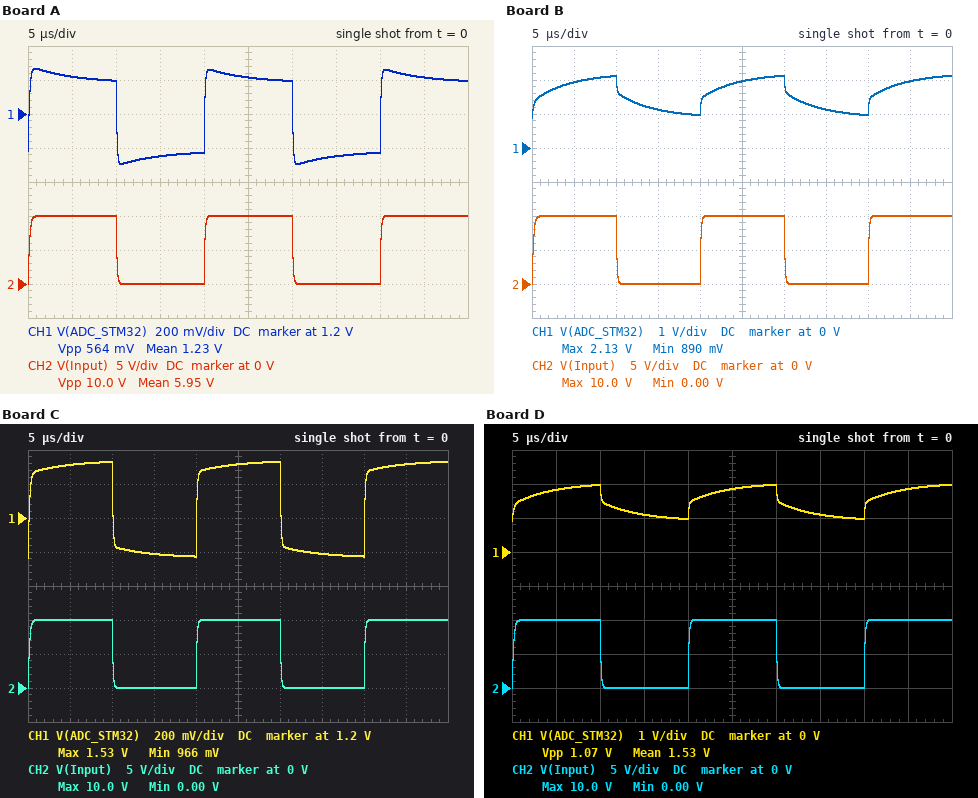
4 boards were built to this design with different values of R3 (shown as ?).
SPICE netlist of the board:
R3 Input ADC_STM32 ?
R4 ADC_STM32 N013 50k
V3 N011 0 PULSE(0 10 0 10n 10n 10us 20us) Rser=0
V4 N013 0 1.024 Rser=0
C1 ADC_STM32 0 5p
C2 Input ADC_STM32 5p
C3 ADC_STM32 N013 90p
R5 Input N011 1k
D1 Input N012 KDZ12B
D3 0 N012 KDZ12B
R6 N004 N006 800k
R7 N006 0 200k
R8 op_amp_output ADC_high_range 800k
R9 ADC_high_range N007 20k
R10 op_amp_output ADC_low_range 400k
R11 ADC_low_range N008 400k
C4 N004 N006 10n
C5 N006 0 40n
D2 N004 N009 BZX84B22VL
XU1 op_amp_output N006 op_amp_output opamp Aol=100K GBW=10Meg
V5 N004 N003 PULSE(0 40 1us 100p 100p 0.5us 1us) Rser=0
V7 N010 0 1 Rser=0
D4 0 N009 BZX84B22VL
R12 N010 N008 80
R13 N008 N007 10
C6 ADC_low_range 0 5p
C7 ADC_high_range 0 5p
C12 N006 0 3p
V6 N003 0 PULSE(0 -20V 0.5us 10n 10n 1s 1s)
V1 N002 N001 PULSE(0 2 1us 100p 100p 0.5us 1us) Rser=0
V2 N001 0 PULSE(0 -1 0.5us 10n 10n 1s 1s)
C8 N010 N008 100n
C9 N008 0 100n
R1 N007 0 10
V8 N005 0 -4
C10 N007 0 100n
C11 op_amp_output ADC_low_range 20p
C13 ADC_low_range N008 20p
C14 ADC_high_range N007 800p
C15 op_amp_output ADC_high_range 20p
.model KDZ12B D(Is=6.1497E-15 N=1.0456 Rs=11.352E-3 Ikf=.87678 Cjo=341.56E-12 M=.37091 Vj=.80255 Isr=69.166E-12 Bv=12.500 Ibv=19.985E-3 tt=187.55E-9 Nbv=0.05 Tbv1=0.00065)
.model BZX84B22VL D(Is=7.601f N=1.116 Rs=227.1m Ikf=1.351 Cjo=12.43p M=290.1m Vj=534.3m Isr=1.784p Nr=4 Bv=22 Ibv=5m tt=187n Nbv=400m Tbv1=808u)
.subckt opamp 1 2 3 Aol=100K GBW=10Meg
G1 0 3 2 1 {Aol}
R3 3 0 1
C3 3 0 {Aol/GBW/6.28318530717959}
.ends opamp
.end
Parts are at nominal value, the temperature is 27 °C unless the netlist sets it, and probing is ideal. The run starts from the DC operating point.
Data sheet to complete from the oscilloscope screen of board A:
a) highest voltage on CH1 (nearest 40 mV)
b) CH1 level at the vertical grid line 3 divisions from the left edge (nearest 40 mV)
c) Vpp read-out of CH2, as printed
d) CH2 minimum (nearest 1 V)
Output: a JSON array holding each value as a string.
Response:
["1.48 V", "960 mV", "10.0 V", "0 V"]
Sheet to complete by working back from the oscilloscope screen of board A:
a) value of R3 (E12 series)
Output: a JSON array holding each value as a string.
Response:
["1.2 MΩ"]
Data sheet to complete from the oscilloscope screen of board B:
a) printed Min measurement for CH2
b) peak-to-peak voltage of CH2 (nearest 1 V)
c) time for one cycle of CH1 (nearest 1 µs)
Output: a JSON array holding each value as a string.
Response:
["0.00 V", "10 V", "20 µs"]
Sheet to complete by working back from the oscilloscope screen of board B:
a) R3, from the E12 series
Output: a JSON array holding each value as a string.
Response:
["330 kΩ"]
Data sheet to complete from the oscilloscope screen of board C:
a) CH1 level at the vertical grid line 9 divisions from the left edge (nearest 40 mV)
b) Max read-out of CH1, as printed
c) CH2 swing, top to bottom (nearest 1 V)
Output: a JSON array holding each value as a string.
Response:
["1.52 V", "1.53 V", "10 V"]
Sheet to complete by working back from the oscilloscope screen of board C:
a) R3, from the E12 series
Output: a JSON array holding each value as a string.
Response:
["820 kΩ"]
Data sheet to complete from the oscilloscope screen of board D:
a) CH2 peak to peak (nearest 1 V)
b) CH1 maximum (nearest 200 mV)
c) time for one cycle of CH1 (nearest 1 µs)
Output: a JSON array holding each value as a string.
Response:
["10 V", "2.0 V", "20 µs"]
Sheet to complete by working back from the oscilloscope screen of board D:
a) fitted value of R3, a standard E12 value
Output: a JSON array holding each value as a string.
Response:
["390 kΩ"]
